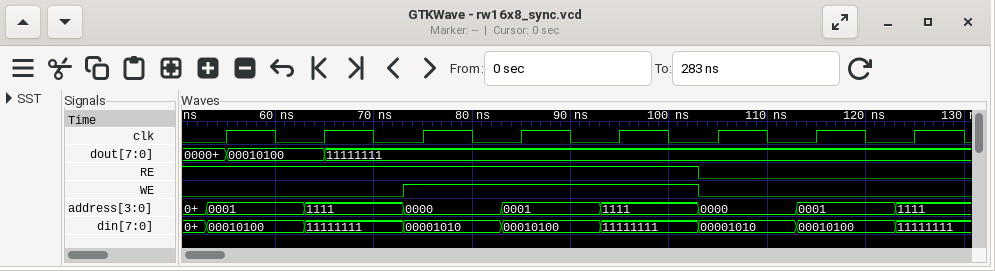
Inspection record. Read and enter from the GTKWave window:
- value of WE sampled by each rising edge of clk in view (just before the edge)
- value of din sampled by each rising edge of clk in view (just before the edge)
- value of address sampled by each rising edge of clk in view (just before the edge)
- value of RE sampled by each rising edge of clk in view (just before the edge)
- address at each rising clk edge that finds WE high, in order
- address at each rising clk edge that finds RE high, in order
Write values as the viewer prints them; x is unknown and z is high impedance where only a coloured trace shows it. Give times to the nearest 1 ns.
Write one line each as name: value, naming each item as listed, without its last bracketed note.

value of WE sampled by each rising edge of clk in view: 0 0 1 1 1 0 0 0
value of din sampled by each rising edge of clk in view: 00010100, 11111111, 00001010, 00010100, 11111111, 00001010, 00010100, 11111111
value of address sampled by each rising edge of clk in view: 0001, 1111, 0000, 0001, 1111, 0000, 0001, 1111
value of RE sampled by each rising edge of clk in view: 1 1 1 1 1 0 0 0
address at each rising clk edge that finds WE high, in order: 0000, 0001, 1111
address at each rising clk edge that finds RE high, in order: 0001, 1111, 0000, 0001, 1111
